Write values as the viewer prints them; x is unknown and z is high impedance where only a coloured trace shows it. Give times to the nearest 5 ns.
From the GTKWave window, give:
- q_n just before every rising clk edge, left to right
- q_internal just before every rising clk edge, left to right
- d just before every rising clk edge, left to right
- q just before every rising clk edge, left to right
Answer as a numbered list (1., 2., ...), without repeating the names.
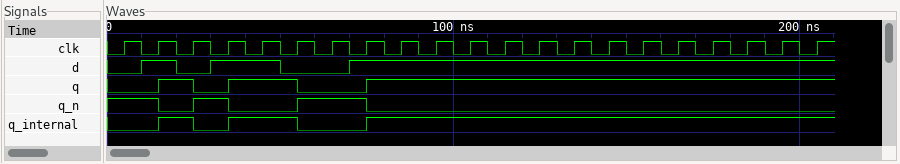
1. 1 1 0 1 0 0 1 1 0 0 0 0 0 0 0 0 0 0 0 0 0
2. 0 0 1 0 1 1 0 0 1 1 1 1 1 1 1 1 1 1 1 1 1
3. 0 1 0 1 1 0 0 1 1 1 1 1 1 1 1 1 1 1 1 1 1
4. 0 0 1 0 1 1 0 0 1 1 1 1 1 1 1 1 1 1 1 1 1
